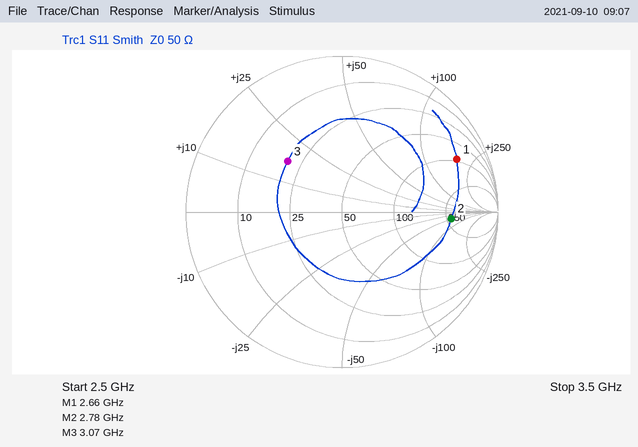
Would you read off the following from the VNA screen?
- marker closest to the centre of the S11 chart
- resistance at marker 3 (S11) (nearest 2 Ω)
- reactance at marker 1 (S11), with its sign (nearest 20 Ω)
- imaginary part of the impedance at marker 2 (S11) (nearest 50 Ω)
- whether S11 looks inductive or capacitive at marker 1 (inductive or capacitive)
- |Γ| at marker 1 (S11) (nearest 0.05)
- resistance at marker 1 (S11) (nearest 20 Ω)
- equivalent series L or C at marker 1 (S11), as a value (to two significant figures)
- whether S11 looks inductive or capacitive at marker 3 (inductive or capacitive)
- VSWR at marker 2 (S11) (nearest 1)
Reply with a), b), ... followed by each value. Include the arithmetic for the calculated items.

a) marker 3
b) 20 Ω
c) +180 Ω
d) -50 Ω
e) inductive
f) 0.80
g) 100 Ω
h) L = 180 Ω/(2π × 2.66 GHz) ≈ 11 nH
i) inductive
j) 6
